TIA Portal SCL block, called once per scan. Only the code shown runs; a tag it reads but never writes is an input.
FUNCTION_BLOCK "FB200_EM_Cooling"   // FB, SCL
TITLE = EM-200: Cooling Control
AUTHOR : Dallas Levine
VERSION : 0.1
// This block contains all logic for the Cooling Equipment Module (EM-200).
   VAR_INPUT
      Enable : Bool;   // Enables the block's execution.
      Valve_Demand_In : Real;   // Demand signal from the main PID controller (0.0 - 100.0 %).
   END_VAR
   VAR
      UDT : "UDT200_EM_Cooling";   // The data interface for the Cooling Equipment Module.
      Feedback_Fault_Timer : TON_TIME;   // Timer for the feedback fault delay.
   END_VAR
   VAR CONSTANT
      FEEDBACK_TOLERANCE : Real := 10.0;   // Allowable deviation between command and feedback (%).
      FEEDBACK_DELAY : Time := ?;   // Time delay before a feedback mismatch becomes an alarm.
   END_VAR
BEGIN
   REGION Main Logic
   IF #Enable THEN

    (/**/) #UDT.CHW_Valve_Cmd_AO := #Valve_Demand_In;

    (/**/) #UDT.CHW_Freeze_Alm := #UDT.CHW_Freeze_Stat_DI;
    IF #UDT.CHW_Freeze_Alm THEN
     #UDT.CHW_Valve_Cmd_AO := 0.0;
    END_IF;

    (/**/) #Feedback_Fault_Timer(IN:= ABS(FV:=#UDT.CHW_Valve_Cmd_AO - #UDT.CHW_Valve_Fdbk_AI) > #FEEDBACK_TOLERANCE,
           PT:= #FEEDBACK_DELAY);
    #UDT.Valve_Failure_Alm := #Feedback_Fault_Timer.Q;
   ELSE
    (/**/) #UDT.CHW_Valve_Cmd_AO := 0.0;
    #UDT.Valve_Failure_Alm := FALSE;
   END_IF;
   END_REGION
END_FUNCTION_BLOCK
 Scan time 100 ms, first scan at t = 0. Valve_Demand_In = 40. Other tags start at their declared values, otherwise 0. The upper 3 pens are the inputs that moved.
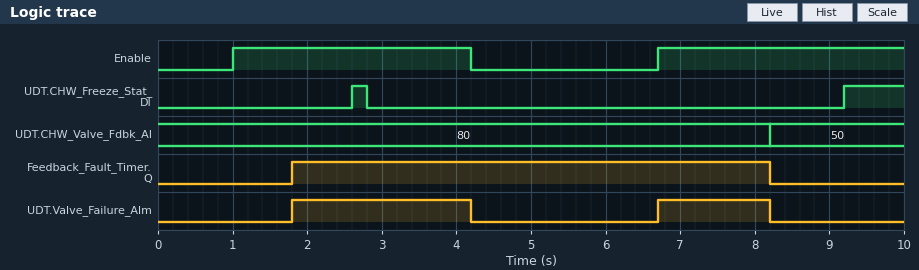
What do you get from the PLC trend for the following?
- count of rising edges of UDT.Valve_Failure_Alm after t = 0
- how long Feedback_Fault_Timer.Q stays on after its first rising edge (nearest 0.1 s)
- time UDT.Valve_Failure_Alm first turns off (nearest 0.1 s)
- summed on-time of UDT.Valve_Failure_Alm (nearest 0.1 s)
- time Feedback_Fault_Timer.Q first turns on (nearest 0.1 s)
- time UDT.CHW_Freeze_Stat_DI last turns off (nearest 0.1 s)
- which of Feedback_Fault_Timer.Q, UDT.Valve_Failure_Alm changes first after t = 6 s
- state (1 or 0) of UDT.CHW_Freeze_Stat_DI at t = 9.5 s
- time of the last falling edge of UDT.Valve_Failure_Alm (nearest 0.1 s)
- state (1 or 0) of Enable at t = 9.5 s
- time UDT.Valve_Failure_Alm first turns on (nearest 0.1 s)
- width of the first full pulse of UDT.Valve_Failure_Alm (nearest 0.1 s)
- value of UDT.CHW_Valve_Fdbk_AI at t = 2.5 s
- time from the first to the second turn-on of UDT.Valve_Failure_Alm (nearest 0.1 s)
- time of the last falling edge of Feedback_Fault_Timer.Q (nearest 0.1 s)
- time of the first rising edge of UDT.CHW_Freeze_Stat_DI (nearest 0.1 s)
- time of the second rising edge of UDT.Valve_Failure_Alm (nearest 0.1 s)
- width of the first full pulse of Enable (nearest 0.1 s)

2
6.4 s
4.2 s
3.9 s
1.8 s
2.8 s
UDT.Valve_Failure_Alm
1
8.2 s
1
1.8 s
2.4 s
80
4.9 s
8.2 s
2.6 s
6.7 s
3.2 s
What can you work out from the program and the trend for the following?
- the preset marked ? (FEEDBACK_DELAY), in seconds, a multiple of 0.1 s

0.8 s
